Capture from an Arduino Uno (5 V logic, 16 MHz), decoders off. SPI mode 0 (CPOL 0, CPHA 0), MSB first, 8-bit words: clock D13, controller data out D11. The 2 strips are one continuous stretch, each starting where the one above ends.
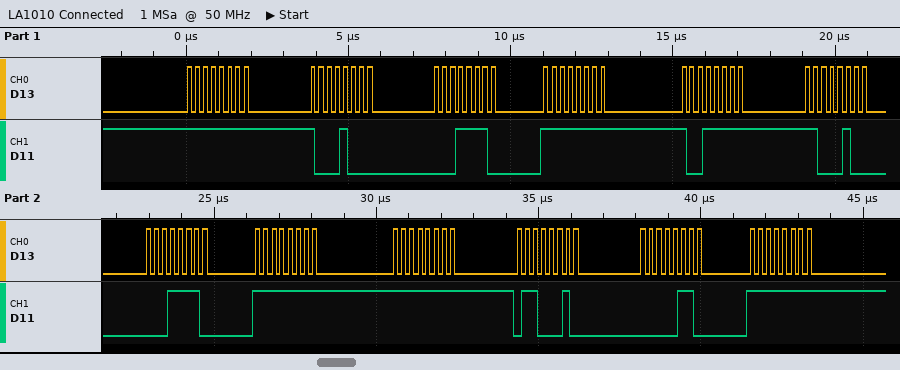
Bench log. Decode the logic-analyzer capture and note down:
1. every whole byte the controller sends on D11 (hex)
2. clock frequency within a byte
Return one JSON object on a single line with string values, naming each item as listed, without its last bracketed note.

{"every whole byte the controller sends on D11": "0xFF 0x88 0x1E 0xFF 0x9F 0xC4 0x1E 0xFF 0xFF 0x62 0x06 0xFF", "clock frequency within a byte": "4 MHz"}
